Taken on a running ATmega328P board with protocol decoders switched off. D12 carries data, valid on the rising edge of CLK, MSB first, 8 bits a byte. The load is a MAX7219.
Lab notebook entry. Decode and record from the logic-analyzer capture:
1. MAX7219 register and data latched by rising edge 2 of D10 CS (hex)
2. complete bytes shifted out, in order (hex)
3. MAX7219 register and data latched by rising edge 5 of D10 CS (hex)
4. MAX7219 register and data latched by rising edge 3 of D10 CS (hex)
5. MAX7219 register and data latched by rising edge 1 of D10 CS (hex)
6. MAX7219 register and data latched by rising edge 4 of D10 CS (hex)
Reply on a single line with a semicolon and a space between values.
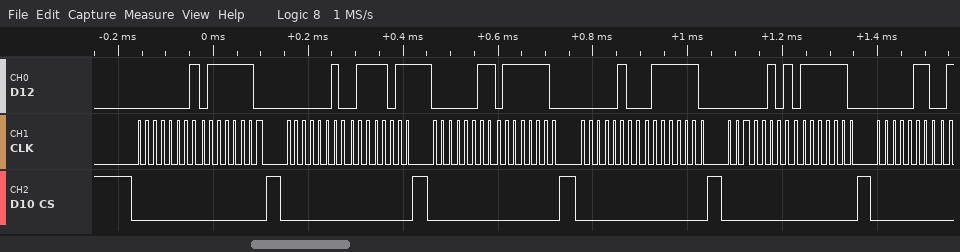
register 0x2, data 0x7B; 01 7E 02 7B 03 7E 04 7E 05 7E 06; register 0x5, data 0x7E; register 0x3, data 0x7E; register 0x1, data 0x7E; register 0x4, data 0x7E
